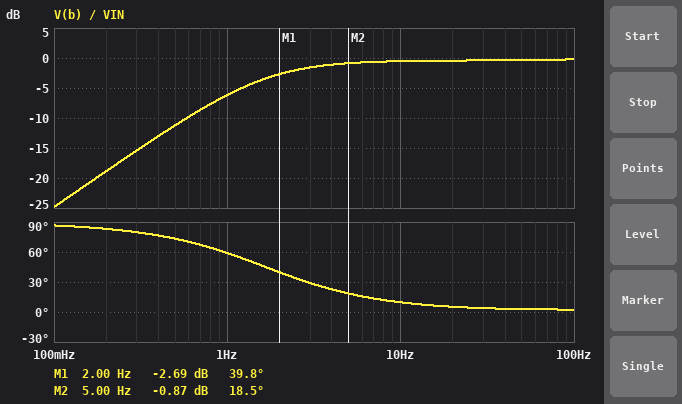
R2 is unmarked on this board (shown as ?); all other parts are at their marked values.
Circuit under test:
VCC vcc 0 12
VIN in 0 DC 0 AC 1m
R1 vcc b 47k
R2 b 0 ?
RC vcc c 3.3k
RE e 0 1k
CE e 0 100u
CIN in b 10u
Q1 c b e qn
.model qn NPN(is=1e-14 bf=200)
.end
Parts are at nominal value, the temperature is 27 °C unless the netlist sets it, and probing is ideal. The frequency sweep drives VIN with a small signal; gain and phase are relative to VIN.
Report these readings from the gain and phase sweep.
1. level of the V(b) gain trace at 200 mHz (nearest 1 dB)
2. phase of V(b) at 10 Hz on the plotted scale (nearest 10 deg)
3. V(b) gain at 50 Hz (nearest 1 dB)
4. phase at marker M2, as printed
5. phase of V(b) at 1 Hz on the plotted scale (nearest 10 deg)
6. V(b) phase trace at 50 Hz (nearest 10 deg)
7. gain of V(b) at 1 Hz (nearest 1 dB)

-19 dB
10 deg
0 dB
18.5 deg
60 deg
0 deg
-6 dB
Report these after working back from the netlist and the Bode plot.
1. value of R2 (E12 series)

12 kΩ
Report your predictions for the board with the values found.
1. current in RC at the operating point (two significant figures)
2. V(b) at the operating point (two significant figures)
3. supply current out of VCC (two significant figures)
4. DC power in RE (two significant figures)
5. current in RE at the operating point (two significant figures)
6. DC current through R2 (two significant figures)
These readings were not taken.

1.7 mA
2.4 V
1.9 mA
2.9 mW
1.7 mA
200 µA
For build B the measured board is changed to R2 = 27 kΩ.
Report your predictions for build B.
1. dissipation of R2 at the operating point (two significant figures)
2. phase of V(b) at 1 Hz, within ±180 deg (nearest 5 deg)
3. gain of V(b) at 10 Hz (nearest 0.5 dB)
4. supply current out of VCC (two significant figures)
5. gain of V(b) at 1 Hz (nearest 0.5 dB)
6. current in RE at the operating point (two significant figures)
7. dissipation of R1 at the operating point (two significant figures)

450 µW
65 deg
-19.5 dB
2.9 mA
-26.0 dB
2.8 mA
1.5 mW
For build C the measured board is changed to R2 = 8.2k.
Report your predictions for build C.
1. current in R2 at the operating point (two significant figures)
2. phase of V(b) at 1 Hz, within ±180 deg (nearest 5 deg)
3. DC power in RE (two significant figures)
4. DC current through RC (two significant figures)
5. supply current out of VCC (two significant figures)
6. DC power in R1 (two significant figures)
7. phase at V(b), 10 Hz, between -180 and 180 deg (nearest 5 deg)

210 µA
65 deg
1.2 mW
1.1 mA
1.3 mA
2.2 mW
15 deg
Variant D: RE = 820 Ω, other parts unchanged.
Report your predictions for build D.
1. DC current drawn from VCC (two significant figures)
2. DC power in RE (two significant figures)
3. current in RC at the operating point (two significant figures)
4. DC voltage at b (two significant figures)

2.2 mA
3.4 mW
2.0 mA
2.3 V
